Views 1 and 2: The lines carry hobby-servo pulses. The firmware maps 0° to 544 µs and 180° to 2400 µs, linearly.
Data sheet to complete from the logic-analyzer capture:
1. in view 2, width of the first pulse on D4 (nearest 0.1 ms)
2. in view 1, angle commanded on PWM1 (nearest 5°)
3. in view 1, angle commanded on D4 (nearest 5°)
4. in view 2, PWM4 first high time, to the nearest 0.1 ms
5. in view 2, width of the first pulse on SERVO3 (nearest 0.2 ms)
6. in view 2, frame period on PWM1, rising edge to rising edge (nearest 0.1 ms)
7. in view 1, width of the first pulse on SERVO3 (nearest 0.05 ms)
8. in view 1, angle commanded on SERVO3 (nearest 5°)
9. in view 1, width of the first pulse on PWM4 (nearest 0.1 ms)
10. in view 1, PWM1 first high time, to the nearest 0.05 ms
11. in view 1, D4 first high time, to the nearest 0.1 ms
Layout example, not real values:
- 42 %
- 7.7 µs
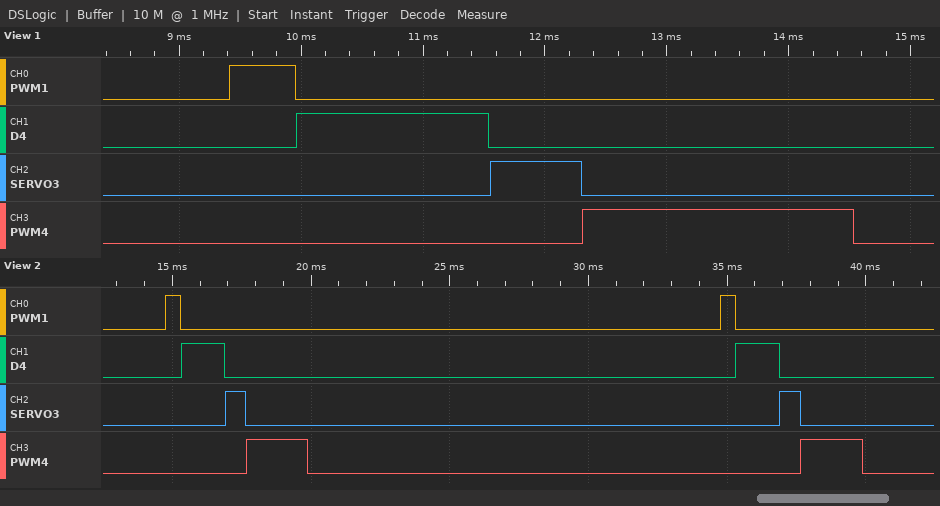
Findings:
- 1.6 ms
- 0°
- 100°
- 2.2 ms
- 0.8 ms
- 20.0 ms
- 0.75 ms
- 20°
- 2.2 ms
- 0.55 ms
- 1.6 ms
